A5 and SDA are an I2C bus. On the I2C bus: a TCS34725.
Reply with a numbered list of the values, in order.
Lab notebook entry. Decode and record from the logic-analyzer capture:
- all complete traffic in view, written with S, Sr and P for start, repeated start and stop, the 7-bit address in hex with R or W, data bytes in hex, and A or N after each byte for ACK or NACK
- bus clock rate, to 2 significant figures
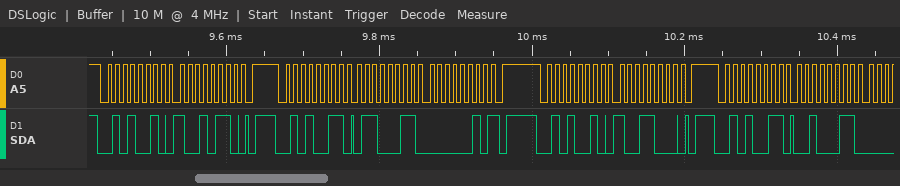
1. S 29W A 96 A P S 29R A 63 A 02 N P S 29W A 98 A P S 29R A 23 A
2. 100 kHz
